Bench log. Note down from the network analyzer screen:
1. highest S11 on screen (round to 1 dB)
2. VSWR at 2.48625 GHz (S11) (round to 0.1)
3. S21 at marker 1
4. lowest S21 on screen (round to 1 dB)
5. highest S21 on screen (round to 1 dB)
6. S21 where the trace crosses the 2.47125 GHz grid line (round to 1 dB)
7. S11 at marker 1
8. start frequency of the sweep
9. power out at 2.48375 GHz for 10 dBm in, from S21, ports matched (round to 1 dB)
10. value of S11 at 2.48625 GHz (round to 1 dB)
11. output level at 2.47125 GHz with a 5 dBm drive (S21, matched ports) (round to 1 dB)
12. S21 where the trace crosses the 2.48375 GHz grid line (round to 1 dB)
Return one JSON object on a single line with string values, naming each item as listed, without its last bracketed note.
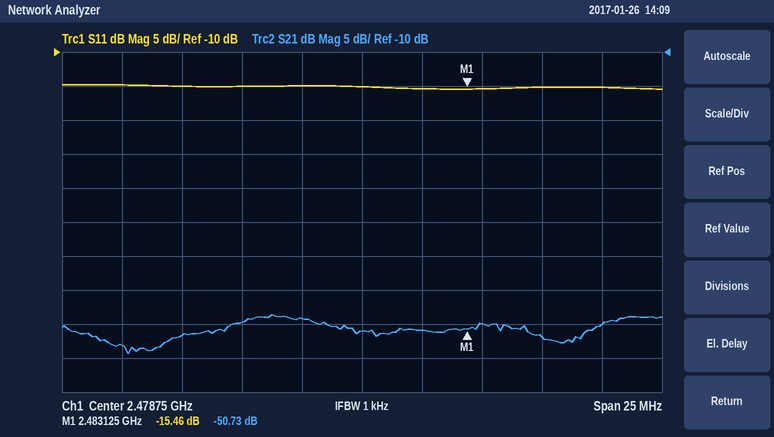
{"highest S11 on screen": "-15 dB", "VSWR at 2.48625 GHz (S11)": "1.4", "S21 at marker 1": "-50.73 dB", "lowest S21 on screen": "-54 dB", "highest S21 on screen": "-49 dB", "S21 where the trace crosses the 2.47125 GHz grid line": "-52 dB", "S11 at marker 1": "-15.46 dB", "start frequency of the sweep": "2.46625 GHz", "power out at 2.48375 GHz for 10 dBm in, from S21, ports matched": "-40 dBm", "value of S11 at 2.48625 GHz": "-15 dB", "output level at 2.47125 GHz with a 5 dBm drive (S21, matched ports)": "-47 dBm", "S21 where the trace crosses the 2.48375 GHz grid line": "-50 dB"}
